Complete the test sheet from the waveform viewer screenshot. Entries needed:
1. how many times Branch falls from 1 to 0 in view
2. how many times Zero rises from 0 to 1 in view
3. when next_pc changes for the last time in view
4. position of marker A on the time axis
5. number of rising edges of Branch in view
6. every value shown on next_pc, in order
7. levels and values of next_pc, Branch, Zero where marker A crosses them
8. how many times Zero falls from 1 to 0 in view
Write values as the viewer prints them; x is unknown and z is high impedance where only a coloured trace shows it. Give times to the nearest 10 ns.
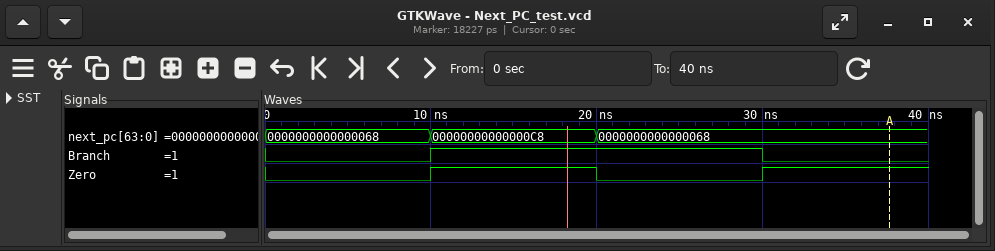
1
2
20 ns
40 ns
1
0000000000000068, 00000000000000C8, 0000000000000068
next_pc=0000000000000068, Branch=0, Zero=1
1
